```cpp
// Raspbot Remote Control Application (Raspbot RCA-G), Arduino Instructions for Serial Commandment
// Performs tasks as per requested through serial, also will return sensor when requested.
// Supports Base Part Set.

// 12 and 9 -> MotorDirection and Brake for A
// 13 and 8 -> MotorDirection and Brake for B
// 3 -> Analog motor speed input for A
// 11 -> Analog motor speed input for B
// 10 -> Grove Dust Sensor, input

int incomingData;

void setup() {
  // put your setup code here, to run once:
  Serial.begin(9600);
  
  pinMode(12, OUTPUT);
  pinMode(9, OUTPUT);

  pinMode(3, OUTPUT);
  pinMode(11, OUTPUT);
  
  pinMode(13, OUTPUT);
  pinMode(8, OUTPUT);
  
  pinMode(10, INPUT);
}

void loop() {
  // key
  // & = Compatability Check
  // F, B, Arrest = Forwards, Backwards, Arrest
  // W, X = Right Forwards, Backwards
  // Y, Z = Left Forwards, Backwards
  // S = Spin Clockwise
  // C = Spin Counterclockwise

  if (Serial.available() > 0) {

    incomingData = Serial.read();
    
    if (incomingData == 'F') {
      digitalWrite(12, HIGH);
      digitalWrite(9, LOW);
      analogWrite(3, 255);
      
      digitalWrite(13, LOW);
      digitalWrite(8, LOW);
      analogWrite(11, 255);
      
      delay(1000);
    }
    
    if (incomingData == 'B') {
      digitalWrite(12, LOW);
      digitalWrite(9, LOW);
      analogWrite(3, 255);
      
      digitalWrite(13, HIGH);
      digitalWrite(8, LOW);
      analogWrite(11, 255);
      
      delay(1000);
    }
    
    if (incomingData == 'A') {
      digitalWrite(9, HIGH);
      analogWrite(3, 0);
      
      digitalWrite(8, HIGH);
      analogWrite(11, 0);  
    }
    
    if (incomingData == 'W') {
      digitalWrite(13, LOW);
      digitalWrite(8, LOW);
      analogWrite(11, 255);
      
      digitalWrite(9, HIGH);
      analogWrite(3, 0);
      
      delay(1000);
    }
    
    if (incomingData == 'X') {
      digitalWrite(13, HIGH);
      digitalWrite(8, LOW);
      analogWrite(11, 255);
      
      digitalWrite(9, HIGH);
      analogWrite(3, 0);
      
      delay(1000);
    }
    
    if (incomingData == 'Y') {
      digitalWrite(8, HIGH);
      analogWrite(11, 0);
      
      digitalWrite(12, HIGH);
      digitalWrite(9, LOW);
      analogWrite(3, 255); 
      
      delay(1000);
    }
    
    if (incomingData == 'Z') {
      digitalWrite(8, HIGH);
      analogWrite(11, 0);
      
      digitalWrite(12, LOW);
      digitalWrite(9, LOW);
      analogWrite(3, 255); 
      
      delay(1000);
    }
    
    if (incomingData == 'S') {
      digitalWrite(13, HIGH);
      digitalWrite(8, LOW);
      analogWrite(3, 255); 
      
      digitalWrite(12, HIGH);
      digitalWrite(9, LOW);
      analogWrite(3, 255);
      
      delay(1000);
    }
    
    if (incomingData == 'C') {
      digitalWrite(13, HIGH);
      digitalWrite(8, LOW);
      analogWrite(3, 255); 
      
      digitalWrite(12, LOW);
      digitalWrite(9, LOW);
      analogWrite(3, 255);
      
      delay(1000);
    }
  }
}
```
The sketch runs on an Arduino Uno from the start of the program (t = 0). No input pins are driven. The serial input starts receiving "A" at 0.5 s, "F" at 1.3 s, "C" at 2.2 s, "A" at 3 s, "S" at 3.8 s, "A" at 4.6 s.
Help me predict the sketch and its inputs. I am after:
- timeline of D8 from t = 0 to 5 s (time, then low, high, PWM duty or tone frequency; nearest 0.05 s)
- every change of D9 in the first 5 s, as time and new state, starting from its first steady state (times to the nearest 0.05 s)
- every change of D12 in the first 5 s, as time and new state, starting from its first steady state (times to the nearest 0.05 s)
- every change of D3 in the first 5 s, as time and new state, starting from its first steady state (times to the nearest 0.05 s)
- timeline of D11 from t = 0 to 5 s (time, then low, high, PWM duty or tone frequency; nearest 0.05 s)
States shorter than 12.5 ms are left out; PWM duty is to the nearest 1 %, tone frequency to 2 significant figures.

0 s low; 0.5 s high; 1.3 s low; 3.3 s high; 3.8 s low; 4.8 s high
0 s low; 0.5 s high; 1.3 s low; 3.3 s high; 3.8 s low; 4.8 s high
0 s low; 1.3 s high; 2.3 s low; 3.8 s high
0 s low; 1.3 s high; 3.3 s low; 3.8 s high; 4.8 s low
0 s low; 1.3 s high; 3.3 s low
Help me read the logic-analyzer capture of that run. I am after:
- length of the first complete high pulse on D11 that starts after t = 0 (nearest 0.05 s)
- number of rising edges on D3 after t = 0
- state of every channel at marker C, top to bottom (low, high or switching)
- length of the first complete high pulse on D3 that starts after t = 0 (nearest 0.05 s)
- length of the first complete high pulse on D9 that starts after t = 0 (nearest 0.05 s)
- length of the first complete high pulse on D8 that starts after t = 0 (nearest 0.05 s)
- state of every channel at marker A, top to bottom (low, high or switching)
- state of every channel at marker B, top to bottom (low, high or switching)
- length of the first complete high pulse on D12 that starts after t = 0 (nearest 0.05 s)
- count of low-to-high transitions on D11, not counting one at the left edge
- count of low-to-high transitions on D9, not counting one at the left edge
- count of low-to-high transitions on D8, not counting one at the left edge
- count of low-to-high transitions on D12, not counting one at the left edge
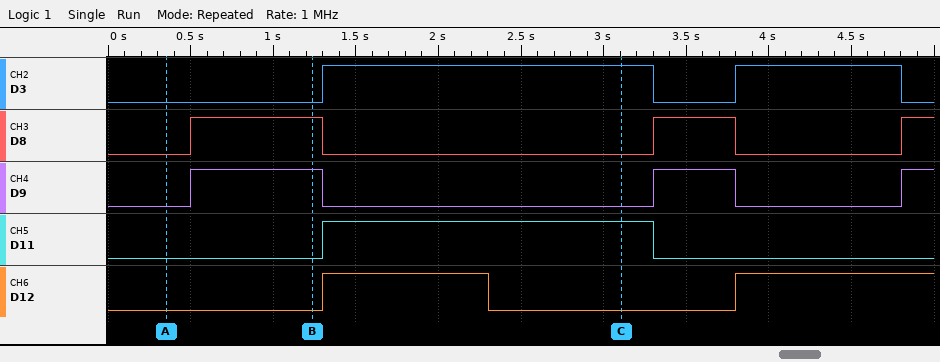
2.00 s
2
D3 high, D8 low, D9 low, D11 high, D12 low
2.00 s
0.80 s
0.80 s
D3 low, D8 low, D9 low, D11 low, D12 low
D3 low, D8 high, D9 high, D11 low, D12 low
1.00 s
1
3
3
2
